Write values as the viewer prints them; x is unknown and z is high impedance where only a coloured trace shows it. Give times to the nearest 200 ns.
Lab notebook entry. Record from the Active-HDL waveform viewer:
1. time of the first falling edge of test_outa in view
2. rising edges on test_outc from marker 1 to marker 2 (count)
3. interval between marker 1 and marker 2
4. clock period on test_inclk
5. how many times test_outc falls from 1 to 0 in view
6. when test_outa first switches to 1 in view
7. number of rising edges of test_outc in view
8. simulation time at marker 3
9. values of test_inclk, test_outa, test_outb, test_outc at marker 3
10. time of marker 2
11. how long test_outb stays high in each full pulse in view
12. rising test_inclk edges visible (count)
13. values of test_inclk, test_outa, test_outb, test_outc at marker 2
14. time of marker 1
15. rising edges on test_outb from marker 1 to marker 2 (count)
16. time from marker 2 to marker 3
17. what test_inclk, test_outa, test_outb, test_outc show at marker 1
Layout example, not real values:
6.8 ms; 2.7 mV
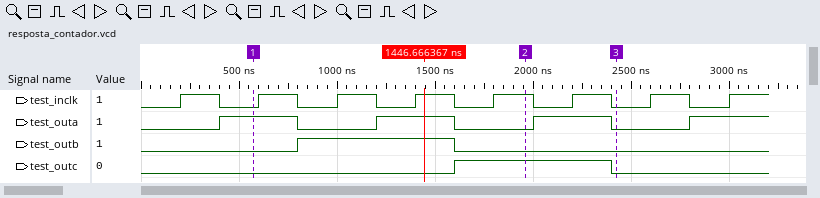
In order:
800 ns; 1; 1400 ns; 400 ns; 1; 400 ns; 1; 2400 ns; test_inclk=0, test_outa=0, test_outb=0, test_outc=0; 2000 ns; 800 ns; 8; test_inclk=1, test_outa=0, test_outb=0, test_outc=1; 600 ns; 1; 400 ns; test_inclk=0, test_outa=1, test_outb=0, test_outc=0
